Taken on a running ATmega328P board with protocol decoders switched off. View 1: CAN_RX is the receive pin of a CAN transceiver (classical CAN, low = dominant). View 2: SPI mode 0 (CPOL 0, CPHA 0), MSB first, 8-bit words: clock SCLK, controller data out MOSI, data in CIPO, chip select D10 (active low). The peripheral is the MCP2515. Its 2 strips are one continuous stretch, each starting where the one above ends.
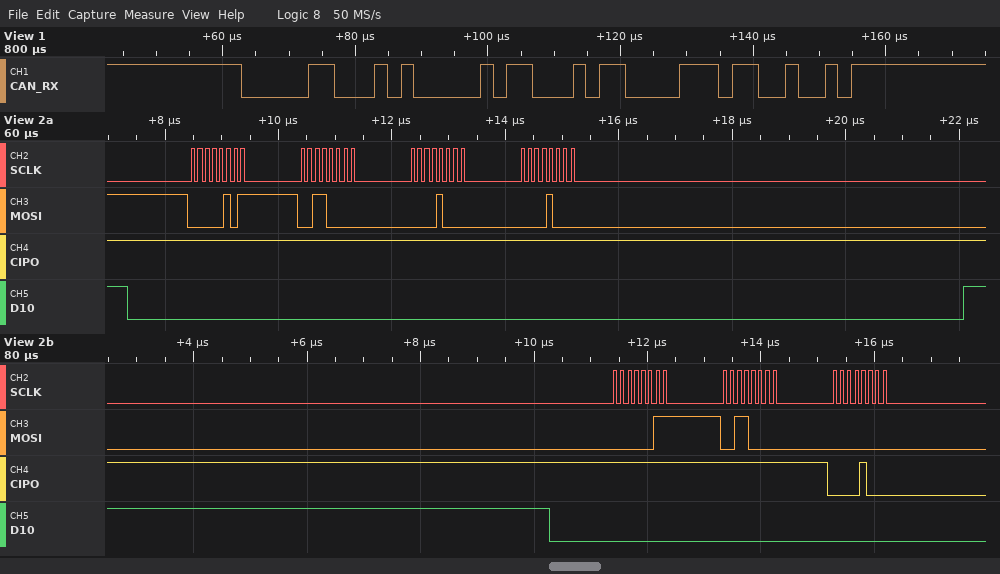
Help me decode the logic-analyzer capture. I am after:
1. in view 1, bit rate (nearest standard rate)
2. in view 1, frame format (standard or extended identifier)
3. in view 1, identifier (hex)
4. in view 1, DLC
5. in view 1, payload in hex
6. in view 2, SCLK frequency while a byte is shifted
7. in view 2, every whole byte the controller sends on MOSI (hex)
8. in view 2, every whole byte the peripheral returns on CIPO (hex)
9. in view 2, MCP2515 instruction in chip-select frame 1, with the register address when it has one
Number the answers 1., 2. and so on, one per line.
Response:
1. 500 kbit/s
2. standard
3. 0x045
4. 1
5. 8B
6. 8 MHz
7. 05 30 08 08 03 30 00
8. FF FF FF FF FF FF 08
9. BIT MODIFY 0x30
